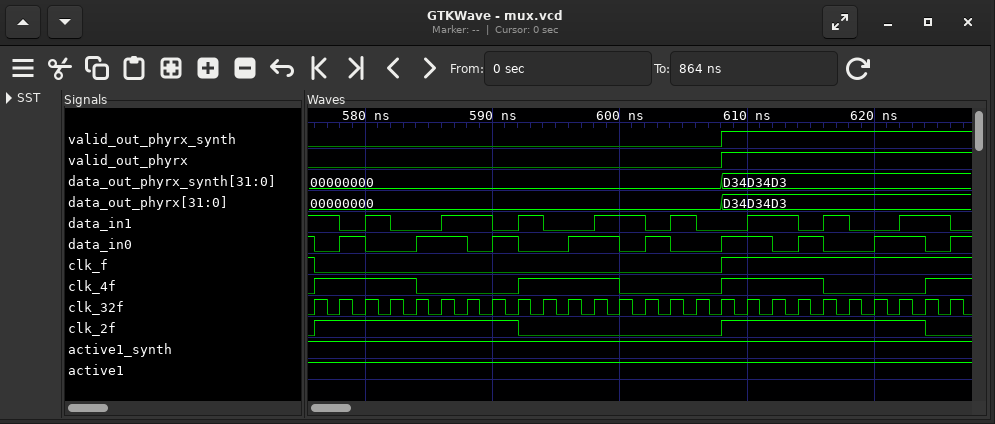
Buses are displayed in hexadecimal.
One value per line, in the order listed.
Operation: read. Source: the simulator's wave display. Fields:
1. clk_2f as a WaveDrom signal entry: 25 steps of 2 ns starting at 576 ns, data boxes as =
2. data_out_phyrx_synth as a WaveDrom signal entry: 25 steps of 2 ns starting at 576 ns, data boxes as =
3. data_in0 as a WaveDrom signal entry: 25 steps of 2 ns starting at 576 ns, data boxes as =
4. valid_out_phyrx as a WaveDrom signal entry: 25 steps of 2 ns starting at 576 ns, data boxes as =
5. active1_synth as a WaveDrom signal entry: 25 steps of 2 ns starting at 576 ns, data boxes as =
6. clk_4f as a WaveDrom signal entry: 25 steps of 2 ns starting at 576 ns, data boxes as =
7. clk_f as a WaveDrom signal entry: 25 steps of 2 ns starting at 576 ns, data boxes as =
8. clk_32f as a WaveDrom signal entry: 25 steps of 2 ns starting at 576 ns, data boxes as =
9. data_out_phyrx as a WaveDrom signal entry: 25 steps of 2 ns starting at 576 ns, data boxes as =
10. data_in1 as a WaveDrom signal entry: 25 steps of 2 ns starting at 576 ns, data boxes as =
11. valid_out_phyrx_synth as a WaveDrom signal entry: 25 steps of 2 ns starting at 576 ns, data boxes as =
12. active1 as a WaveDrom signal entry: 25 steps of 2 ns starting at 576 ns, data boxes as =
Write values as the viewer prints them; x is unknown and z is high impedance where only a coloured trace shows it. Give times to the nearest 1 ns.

{name: 'clk_2f', wave: '1.......0.......1.......0'}
{name: 'data_out_phyrx_synth', wave: '=...............=........', data: '00000000 D34D34D3'}
{name: 'data_in0', wave: '010.1.010.1.010.1.010.1.0'}
{name: 'valid_out_phyrx', wave: '0...............1........'}
{name: 'active1_synth', wave: '1........................'}
{name: 'clk_4f', wave: '1...0...1...0...1...0...1'}
{name: 'clk_f', wave: '0...............1........'}
{name: 'clk_32f', wave: 'p........................'}
{name: 'data_out_phyrx', wave: '=...............=........', data: '00000000 D34D34D3'}
{name: 'data_in1', wave: '1010.1.010.1.010.1.010.1.'}
{name: 'valid_out_phyrx_synth', wave: '0...............1........'}
{name: 'active1', wave: '1........................'}
